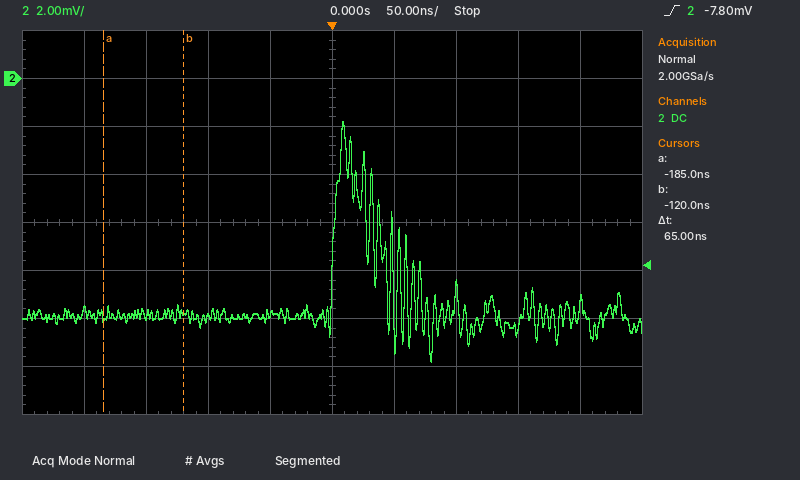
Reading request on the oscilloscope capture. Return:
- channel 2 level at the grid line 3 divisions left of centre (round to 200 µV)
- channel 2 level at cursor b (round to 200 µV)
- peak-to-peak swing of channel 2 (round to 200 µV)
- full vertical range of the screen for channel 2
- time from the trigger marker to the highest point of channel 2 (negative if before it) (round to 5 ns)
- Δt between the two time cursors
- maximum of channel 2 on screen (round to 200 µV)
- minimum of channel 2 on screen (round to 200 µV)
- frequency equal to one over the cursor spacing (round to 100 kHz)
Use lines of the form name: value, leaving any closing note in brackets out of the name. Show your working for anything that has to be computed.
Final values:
channel 2 level at the grid line 3 divisions left of centre: -9.8 mV
channel 2 level at cursor b: -9.8 mV
peak-to-peak swing of channel 2: -1.8 mV − (-11.8 mV) = 10.0 mV
full vertical range of the screen for channel 2: 16 mV
time from the trigger marker to the highest point of channel 2 (negative if before it): +10 ns
Δt between the two time cursors: 65 ns
maximum of channel 2 on screen: -1.8 mV
minimum of channel 2 on screen: -11.8 mV
frequency equal to one over the cursor spacing: 1 / 65 ns ≈ 15.4 MHz
